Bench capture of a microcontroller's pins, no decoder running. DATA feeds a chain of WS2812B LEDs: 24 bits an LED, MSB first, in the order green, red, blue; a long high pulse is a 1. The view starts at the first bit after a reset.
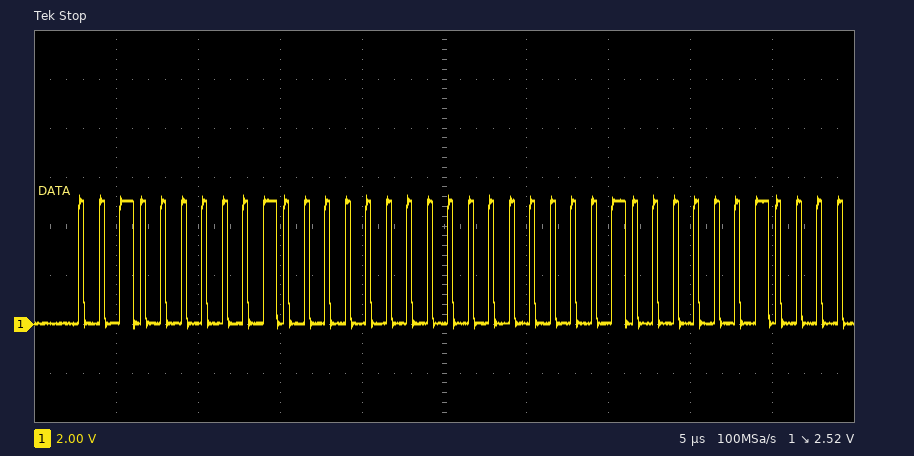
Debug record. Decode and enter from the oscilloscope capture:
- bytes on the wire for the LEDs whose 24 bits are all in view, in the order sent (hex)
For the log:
20 40 00
